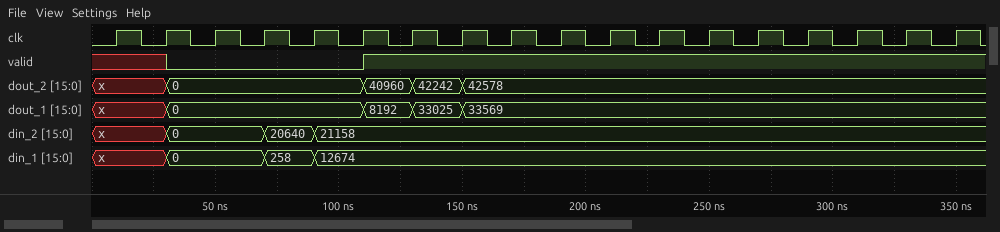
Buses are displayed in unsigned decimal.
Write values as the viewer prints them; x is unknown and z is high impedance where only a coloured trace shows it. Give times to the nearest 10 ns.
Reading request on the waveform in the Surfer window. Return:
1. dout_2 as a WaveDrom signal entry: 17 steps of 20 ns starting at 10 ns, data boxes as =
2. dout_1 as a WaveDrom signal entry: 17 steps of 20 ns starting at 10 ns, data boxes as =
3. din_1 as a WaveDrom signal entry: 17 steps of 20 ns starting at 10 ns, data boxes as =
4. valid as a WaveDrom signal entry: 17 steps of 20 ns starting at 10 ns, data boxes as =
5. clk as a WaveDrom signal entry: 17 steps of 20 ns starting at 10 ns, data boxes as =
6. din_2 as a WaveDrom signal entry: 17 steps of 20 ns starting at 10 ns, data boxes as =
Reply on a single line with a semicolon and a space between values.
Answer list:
{name: 'dout_2', wave: 'x=...===.........', data: '0 40960 42242 42578'}; {name: 'dout_1', wave: 'x=...===.........', data: '0 8192 33025 33569'}; {name: 'din_1', wave: 'x=.==............', data: '0 258 12674'}; {name: 'valid', wave: 'x0...1...........'}; {name: 'clk', wave: 'p................'}; {name: 'din_2', wave: 'x=.==............', data: '0 20640 21158'}
